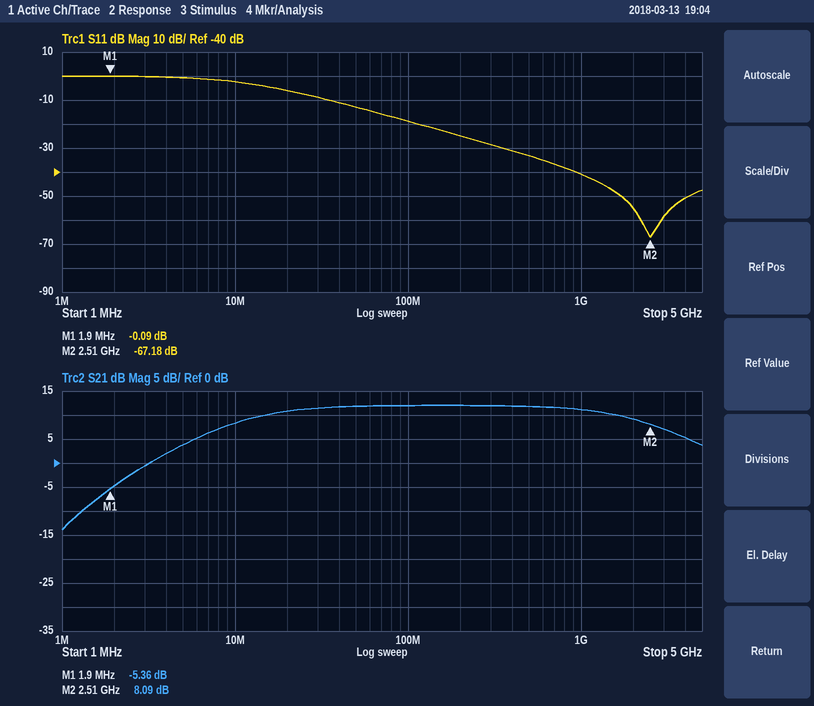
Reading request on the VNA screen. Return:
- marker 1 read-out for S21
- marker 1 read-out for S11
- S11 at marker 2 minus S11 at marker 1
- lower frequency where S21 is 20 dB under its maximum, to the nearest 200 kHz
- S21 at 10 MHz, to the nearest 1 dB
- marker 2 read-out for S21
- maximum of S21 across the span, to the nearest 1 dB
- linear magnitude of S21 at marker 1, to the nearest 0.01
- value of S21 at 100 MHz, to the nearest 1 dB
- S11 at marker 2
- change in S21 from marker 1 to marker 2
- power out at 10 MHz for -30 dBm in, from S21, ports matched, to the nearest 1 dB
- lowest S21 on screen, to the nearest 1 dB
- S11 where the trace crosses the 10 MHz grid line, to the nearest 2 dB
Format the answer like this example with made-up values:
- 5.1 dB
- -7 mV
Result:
- -5.36 dB
- -0.09 dB
- -67.09 dB
- 1.6 MHz
- 8 dB
- 8.09 dB
- 12 dB
- 0.54
- 12 dB
- -67.18 dB
- 13.45 dB
- -22 dBm
- -14 dB
- -2 dB
